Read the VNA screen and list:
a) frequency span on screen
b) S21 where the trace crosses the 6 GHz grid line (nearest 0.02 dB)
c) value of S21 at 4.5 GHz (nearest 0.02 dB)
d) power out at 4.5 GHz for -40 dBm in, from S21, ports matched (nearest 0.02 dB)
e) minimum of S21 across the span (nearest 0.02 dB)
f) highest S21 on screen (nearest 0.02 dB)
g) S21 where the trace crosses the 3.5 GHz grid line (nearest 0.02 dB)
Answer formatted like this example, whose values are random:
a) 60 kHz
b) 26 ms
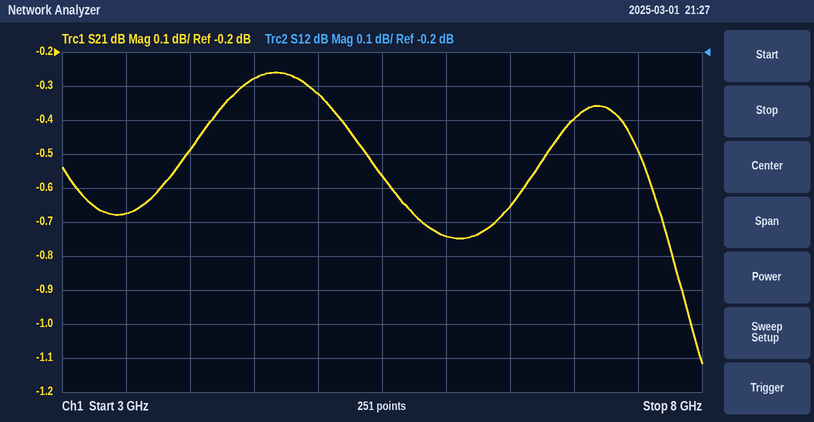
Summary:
a) 5 GHz
b) -0.74 dB
c) -0.28 dB
d) -40.28 dBm
e) -1.12 dB
f) -0.26 dB
g) -0.68 dB
